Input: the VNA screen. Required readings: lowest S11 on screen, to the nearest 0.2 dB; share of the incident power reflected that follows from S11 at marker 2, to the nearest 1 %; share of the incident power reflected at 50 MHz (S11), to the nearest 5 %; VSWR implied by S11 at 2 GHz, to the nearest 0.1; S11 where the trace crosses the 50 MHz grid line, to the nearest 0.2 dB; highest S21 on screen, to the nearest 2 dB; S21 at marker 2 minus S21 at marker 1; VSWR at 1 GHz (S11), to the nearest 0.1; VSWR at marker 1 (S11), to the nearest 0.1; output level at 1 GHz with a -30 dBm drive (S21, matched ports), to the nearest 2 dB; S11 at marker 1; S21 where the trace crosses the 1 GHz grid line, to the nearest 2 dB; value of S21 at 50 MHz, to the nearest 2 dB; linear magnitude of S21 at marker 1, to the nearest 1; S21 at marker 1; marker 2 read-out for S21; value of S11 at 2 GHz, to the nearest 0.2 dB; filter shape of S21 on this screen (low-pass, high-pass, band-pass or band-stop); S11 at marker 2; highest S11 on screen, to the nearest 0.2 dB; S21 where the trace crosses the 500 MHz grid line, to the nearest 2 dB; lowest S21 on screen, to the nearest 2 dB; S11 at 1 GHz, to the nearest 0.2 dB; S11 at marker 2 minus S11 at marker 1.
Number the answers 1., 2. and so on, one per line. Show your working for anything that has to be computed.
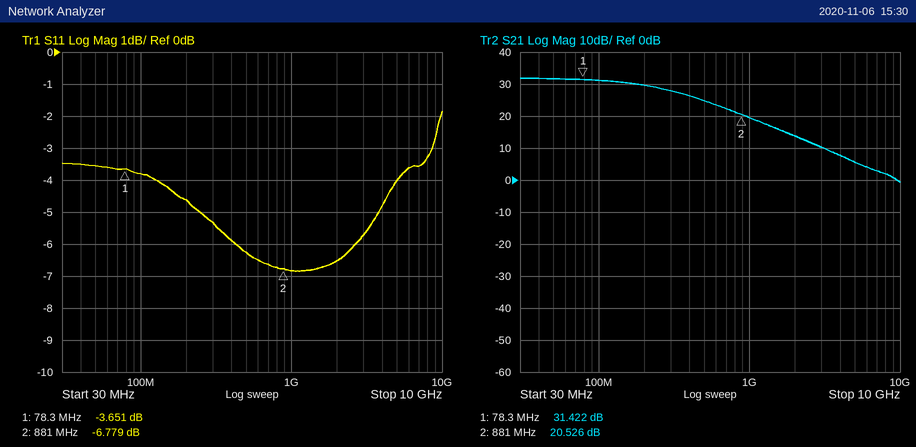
1. -6.8 dB
2. 10^(-6.779/10) ≈ 21 %
3. 10^(-3.6/10) ≈ 43.7 %, so 45 % to the nearest 5 %
4. |Γ| = 10^(-6.6/20) = 0.4677; VSWR = (1 + 0.4677)/(1 − 0.4677) ≈ 2.8
5. -3.6 dB
6. 32 dB
7. 20.526 − (31.422) = -10.896 dB
8. |Γ| = 10^(-6.8/20) = 0.4571; VSWR = (1 + 0.4571)/(1 − 0.4571) ≈ 2.7
9. (1 + 0.6568)/(1 − 0.6568) ≈ 4.8
10. -30 dBm + (20 dB) = -10 dBm
11. -3.651 dB
12. 20 dB
13. 32 dB
14. 10^(31.422/20) ≈ 37
15. 31.422 dB
16. 20.526 dB
17. -6.6 dB
18. low-pass
19. -6.779 dB
20. -1.8 dB
21. 24 dB
22. 0 dB
23. -6.8 dB
24. -6.779 − (-3.651) = -3.128 dB
